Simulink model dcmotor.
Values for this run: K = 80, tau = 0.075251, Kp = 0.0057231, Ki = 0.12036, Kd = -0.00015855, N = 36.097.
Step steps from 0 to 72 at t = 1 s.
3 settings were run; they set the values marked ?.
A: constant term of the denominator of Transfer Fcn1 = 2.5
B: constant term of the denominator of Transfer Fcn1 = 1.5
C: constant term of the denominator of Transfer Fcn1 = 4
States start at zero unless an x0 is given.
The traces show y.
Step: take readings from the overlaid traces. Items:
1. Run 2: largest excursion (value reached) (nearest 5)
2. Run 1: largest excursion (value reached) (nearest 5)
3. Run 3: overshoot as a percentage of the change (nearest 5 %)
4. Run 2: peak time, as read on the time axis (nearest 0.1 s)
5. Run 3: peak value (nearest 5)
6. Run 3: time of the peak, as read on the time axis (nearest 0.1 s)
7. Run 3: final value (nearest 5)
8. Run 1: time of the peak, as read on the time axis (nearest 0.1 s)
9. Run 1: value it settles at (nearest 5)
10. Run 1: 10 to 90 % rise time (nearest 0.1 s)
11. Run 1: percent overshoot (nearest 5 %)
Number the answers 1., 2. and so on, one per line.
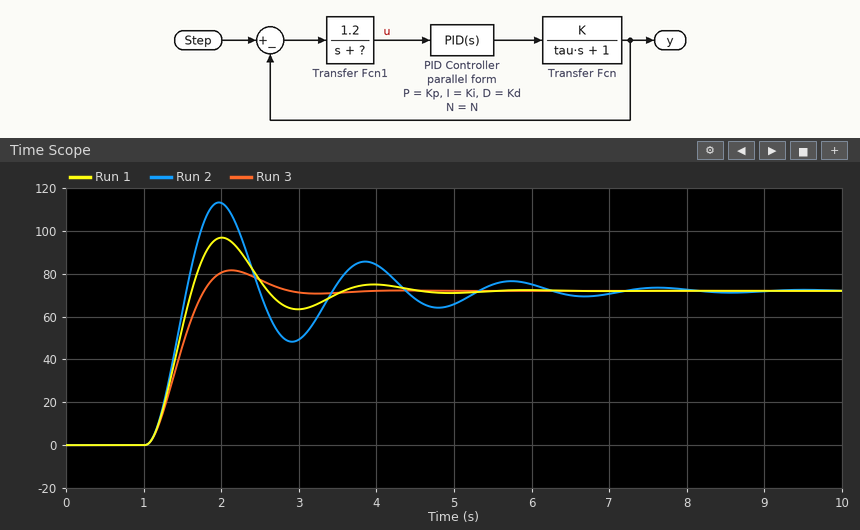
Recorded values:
1. 115
2. 95
3. 15 %
4. 2.0 s
5. 80
6. 2.1 s
7. 70
8. 2.0 s
9. 70
10. 0.4 s
11. 35 %
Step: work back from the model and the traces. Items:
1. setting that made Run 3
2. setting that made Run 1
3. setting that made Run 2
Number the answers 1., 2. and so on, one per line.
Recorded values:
1. C
2. A
3. B
